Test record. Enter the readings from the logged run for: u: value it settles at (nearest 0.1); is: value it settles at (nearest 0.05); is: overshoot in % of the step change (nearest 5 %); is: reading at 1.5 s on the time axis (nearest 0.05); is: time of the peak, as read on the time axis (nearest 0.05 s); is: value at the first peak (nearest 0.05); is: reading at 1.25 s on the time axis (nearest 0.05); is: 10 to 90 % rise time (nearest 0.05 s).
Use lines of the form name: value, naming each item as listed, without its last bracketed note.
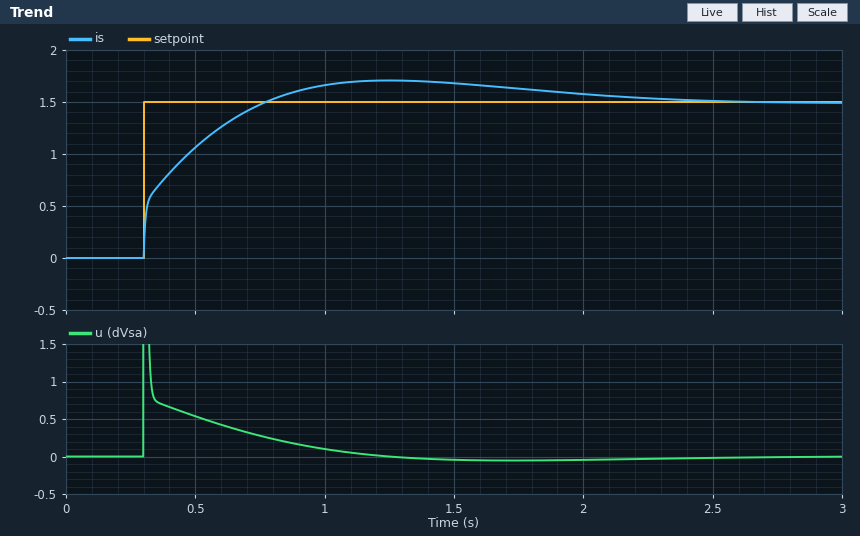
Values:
u: value it settles at: 0.0
is: value it settles at: 1.50
is: overshoot in % of the step change: 15 %
is: reading at 1.5 s on the time axis: 1.70
is: time of the peak, as read on the time axis: 1.25 s
is: value at the first peak: 1.70
is: reading at 1.25 s on the time axis: 1.70
is: 10 to 90 % rise time: 0.35 s
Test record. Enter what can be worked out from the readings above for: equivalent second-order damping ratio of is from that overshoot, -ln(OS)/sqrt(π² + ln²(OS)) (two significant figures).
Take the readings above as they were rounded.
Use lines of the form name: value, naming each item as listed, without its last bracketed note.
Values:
equivalent second-order damping ratio of is from that overshoot, -ln(OS)/sqrt(π² + ln²(OS)): 0.52
